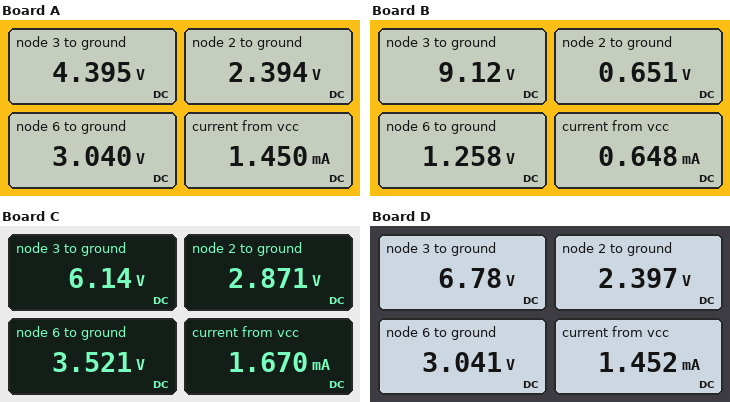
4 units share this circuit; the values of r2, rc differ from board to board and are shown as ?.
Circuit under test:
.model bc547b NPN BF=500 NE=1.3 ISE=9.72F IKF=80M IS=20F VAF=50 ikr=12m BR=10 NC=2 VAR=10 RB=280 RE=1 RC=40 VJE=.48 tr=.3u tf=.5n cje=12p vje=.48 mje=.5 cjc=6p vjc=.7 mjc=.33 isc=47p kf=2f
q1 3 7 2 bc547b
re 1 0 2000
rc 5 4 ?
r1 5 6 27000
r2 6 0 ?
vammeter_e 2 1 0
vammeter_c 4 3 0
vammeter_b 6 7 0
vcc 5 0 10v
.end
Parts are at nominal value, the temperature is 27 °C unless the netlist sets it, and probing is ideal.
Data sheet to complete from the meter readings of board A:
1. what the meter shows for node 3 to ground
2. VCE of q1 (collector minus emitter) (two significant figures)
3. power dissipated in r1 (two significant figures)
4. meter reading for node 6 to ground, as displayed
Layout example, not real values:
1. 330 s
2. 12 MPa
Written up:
1. 4.395 V
2. 2.0 V
3. 1.8 mW
4. 3.040 V
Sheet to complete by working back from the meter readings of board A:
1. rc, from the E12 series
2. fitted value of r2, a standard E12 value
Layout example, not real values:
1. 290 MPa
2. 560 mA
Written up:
1. 4.7 kΩ
2. 12 kΩ
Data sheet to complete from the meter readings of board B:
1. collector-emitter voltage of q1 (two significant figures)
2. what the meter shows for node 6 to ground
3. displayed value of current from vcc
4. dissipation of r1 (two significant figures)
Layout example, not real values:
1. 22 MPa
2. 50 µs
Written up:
1. 8.5 V
2. 1.258 V
3. 0.648 mA
4. 2.8 mW
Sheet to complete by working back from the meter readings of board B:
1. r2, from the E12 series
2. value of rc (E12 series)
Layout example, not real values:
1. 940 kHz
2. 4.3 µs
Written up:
1. 3.9 kΩ
2. 2.7 kΩ
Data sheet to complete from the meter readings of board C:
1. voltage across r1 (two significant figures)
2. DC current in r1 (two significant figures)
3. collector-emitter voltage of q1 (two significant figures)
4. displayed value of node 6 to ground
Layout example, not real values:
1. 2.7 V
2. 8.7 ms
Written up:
1. 6.5 V
2. 240 µA
3. 3.3 V
4. 3.521 V
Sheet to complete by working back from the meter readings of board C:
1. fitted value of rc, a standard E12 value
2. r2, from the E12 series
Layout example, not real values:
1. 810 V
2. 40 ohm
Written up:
1. 2.7 kΩ
2. 15 kΩ
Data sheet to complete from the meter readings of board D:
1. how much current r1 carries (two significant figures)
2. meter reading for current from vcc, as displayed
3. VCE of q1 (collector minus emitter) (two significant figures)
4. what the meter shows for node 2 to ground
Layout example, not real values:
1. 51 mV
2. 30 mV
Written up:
1. 260 µA
2. 1.452 mA
3. 4.4 V
4. 2.397 V
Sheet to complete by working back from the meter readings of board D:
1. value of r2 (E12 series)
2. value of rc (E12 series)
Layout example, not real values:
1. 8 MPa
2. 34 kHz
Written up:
1. 12 kΩ
2. 2.7 kΩ
